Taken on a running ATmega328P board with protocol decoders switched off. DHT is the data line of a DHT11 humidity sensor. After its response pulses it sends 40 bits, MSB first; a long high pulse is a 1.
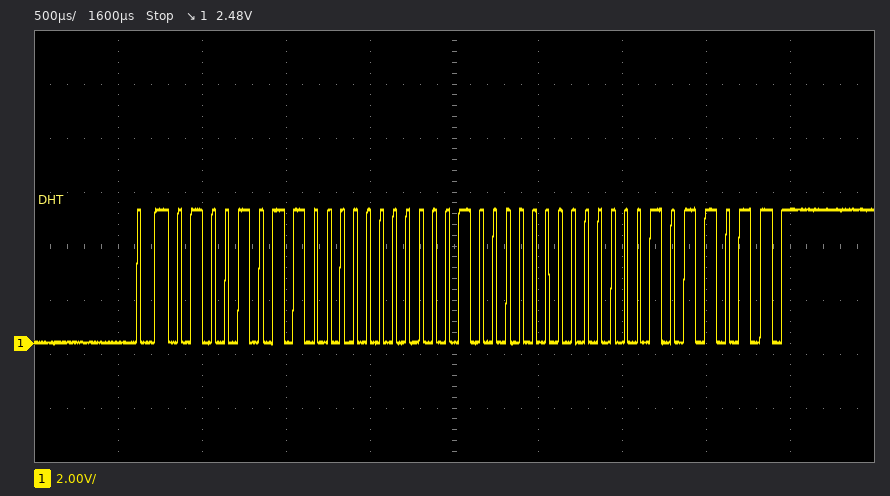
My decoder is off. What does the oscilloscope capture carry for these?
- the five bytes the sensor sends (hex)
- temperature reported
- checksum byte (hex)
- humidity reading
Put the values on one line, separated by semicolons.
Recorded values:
4B 00 10 00 5B; 16.0 °C; 0x5B; 75 %
